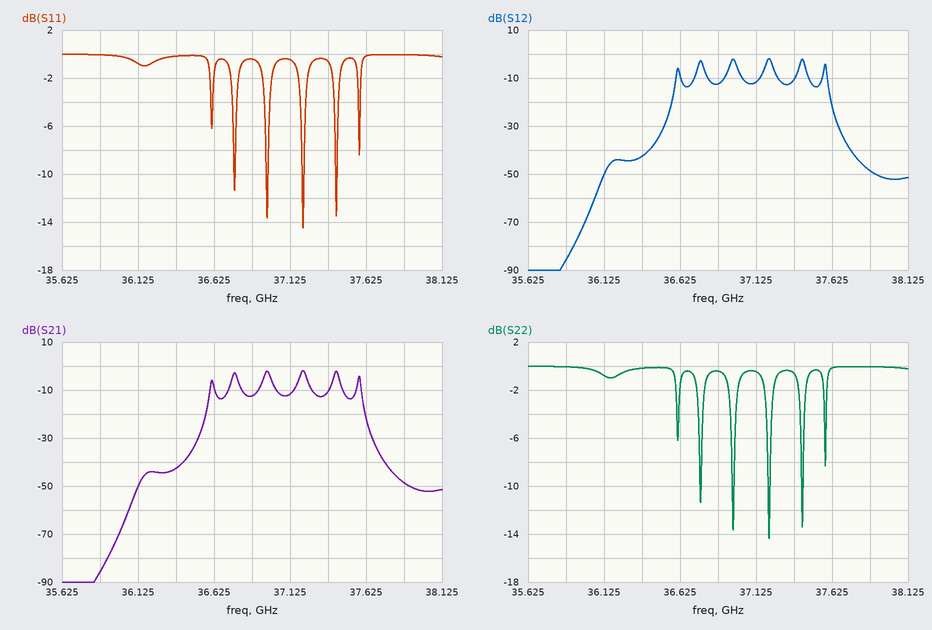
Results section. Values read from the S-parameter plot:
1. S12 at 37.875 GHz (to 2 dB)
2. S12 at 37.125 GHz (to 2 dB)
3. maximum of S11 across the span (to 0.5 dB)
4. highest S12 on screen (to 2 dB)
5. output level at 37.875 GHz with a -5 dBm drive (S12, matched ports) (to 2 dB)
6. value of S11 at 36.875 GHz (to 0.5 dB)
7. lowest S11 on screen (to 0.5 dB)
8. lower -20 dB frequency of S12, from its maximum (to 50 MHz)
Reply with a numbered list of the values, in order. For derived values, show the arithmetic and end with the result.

1. -48 dB
2. -12 dB
3. 0.0 dB
4. -2 dB
5. -5 dBm + (-48 dB) = -54 dBm
6. -0.5 dB
7. -14.5 dB
8. 36.55 GHz
